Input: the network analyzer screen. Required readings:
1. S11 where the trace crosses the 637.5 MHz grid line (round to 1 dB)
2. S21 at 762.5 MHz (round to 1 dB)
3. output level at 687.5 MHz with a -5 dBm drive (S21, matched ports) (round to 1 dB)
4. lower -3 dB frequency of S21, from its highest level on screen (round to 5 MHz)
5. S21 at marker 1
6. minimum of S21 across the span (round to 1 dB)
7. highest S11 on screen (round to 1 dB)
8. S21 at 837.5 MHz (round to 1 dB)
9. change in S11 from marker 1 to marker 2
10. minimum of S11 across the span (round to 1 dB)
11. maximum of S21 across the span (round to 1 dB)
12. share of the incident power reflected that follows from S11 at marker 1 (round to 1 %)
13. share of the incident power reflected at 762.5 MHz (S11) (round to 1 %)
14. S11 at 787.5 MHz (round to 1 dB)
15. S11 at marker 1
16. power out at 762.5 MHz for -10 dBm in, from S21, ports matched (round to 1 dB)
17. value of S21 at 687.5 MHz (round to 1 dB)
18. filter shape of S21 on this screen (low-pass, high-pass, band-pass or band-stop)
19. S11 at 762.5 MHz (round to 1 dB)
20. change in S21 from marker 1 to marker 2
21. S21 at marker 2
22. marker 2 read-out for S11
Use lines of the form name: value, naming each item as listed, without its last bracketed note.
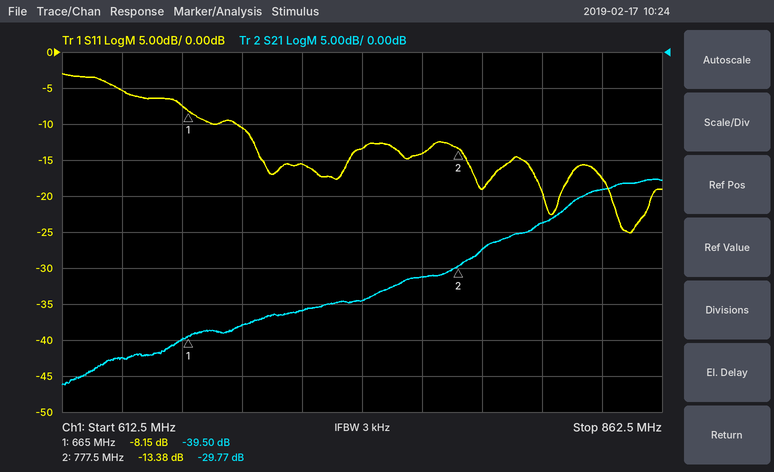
S11 where the trace crosses the 637.5 MHz grid line: -5 dB
S21 at 762.5 MHz: -31 dB
output level at 687.5 MHz with a -5 dBm drive (S21, matched ports): -43 dBm
lower -3 dB frequency of S21, from its highest level on screen: 825 MHz
S21 at marker 1: -39.50 dB
minimum of S21 across the span: -46 dB
highest S11 on screen: -3 dB
S21 at 837.5 MHz: -19 dB
change in S11 from marker 1 to marker 2: -5.23 dB
minimum of S11 across the span: -25 dB
maximum of S21 across the span: -18 dB
share of the incident power reflected that follows from S11 at marker 1: 15 %
share of the incident power reflected at 762.5 MHz (S11): 4 %
S11 at 787.5 MHz: -19 dB
S11 at marker 1: -8.15 dB
power out at 762.5 MHz for -10 dBm in, from S21, ports matched: -41 dBm
value of S21 at 687.5 MHz: -38 dB
filter shape of S21 on this screen: high-pass
S11 at 762.5 MHz: -14 dB
change in S21 from marker 1 to marker 2: 9.73 dB
S21 at marker 2: -29.77 dB
marker 2 read-out for S11: -13.38 dB
